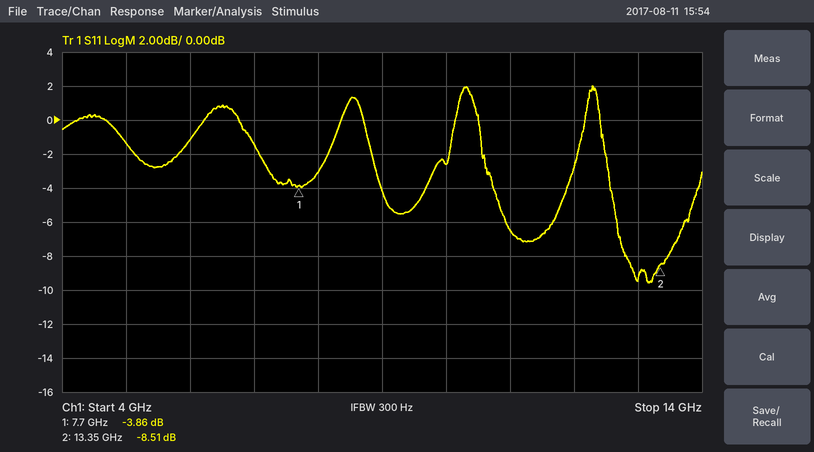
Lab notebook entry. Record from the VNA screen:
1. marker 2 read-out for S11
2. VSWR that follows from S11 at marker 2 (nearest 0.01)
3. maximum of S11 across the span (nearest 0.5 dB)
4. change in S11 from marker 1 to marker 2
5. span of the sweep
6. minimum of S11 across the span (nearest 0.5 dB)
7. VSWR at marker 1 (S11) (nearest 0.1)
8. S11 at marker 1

-8.51 dB
2.20
2.0 dB
-4.65 dB
10 GHz
-9.5 dB
4.6
-3.86 dB
